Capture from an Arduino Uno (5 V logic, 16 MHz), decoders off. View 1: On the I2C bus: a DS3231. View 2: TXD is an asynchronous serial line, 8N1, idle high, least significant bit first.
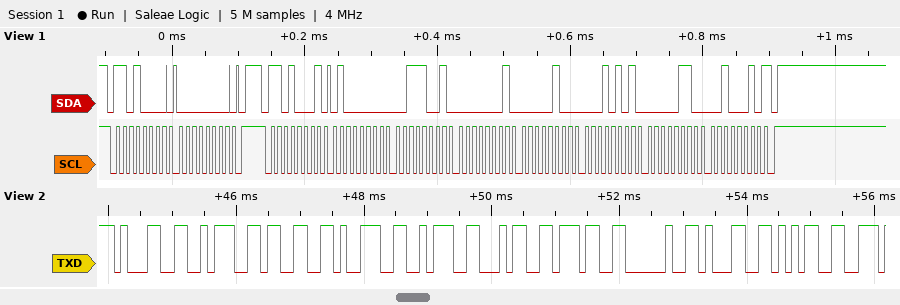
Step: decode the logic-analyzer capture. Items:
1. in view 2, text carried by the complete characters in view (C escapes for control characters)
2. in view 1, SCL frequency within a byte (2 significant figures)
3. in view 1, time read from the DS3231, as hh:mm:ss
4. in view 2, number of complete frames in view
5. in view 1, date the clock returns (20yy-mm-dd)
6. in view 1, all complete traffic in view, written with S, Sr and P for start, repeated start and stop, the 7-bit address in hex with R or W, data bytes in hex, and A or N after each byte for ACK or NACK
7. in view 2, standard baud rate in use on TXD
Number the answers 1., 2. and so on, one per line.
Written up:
1. "1:39:47 15"
2. 100 kHz
3. 01:39:40
4. 10
5. 2022-06-15
6. S 68W A 00 A P S 68R A 40 A 39 A 01 A 04 A 15 A 06 A 22 N P
7. 9600 baud
